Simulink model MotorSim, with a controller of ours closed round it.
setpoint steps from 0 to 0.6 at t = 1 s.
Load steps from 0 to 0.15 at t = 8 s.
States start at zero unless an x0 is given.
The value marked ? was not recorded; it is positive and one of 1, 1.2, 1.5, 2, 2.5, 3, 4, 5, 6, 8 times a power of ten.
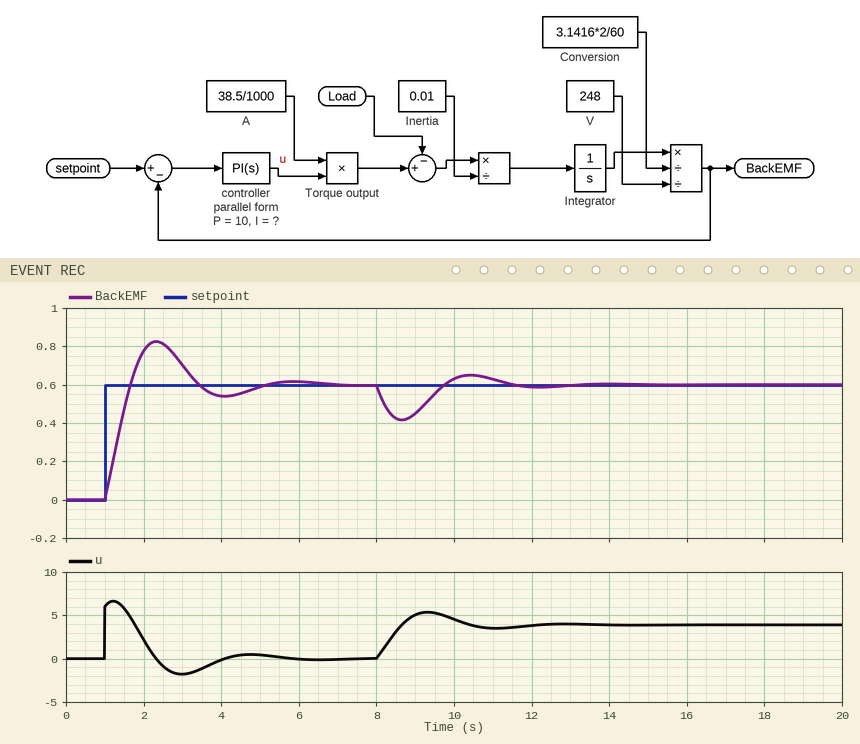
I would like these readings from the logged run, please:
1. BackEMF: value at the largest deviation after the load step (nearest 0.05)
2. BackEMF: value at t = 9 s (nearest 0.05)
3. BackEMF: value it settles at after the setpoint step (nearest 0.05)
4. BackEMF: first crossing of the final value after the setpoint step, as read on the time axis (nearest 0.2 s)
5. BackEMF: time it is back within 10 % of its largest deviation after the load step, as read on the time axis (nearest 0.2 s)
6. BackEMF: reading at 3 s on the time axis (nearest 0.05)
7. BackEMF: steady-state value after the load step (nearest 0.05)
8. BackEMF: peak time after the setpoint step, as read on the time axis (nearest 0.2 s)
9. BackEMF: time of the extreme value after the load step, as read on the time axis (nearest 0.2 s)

0.40
0.45
0.60
1.6 s
11.2 s
0.70
0.60
2.4 s
8.6 s
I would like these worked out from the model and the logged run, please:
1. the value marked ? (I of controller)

25
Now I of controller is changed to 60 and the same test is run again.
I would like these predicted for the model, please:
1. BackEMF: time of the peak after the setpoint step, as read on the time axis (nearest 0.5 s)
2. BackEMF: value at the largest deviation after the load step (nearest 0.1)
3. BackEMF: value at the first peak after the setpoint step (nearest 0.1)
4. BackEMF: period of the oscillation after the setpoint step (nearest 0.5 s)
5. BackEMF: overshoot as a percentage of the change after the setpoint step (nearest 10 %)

2.0 s
0.5
0.9
2.0 s
50 %
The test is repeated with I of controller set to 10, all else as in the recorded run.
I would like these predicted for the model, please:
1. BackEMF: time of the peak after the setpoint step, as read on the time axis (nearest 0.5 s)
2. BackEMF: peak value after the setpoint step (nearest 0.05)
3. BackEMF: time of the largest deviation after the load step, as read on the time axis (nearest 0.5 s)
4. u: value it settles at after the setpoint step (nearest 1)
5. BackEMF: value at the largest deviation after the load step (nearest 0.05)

3.0 s
0.75
9.0 s
0
0.35
